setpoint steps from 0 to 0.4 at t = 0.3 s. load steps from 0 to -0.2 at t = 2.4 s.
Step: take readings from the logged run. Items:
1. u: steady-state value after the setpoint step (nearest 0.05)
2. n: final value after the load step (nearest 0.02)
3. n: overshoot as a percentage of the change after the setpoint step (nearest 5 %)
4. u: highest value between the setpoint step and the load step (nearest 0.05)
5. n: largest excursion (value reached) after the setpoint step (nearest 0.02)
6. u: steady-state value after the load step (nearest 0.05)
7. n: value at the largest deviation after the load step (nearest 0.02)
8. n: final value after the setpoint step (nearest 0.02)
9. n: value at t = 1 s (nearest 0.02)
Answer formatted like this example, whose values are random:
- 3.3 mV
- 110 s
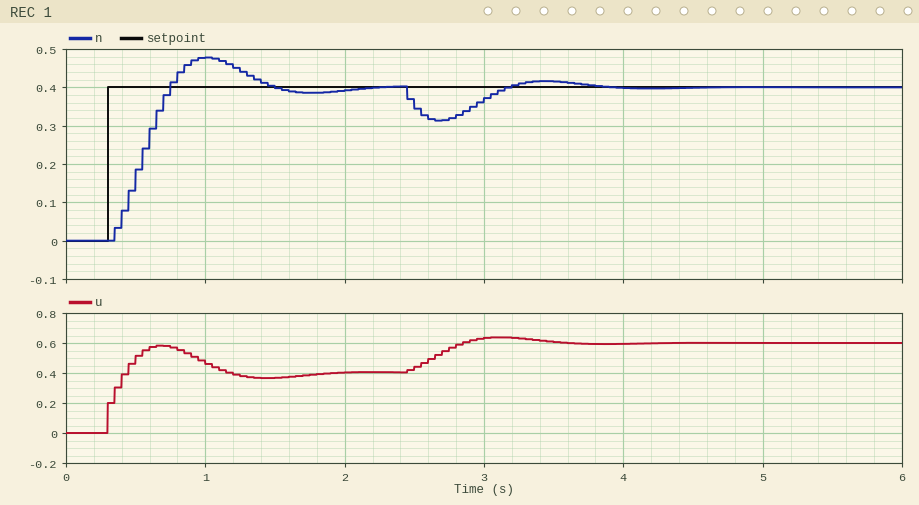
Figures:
- 0.40
- 0.40
- 20 %
- 0.60
- 0.48
- 0.60
- 0.32
- 0.40
- 0.48
